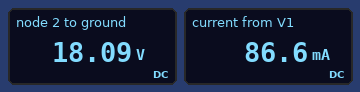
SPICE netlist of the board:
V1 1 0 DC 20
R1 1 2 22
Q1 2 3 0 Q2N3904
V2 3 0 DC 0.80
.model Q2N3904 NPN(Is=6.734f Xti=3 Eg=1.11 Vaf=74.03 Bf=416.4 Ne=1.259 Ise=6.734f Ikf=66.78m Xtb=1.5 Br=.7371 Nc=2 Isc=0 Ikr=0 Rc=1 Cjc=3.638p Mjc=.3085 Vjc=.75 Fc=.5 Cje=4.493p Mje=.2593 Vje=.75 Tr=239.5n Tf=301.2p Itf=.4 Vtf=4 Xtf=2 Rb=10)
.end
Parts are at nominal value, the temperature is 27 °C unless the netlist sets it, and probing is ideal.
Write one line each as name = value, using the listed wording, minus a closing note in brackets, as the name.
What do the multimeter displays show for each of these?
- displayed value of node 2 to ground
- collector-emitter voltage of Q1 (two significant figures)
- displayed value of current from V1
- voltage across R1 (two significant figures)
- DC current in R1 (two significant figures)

displayed value of node 2 to ground = 18.09 V
collector-emitter voltage of Q1 = 18 V
displayed value of current from V1 = 86.6 mA
voltage across R1 = 1.9 V
DC current in R1 = 87 mA
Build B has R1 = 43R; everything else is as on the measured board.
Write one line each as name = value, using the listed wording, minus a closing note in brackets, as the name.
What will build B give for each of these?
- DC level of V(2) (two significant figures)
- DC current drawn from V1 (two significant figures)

DC level of V(2) = 16 V
DC current drawn from V1 = 85 mA
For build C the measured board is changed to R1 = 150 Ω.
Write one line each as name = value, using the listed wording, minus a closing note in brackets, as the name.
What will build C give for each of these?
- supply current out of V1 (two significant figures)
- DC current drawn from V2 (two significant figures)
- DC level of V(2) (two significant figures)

supply current out of V1 = 77 mA
DC current drawn from V2 = 610 µA
DC level of V(2) = 8.4 V
